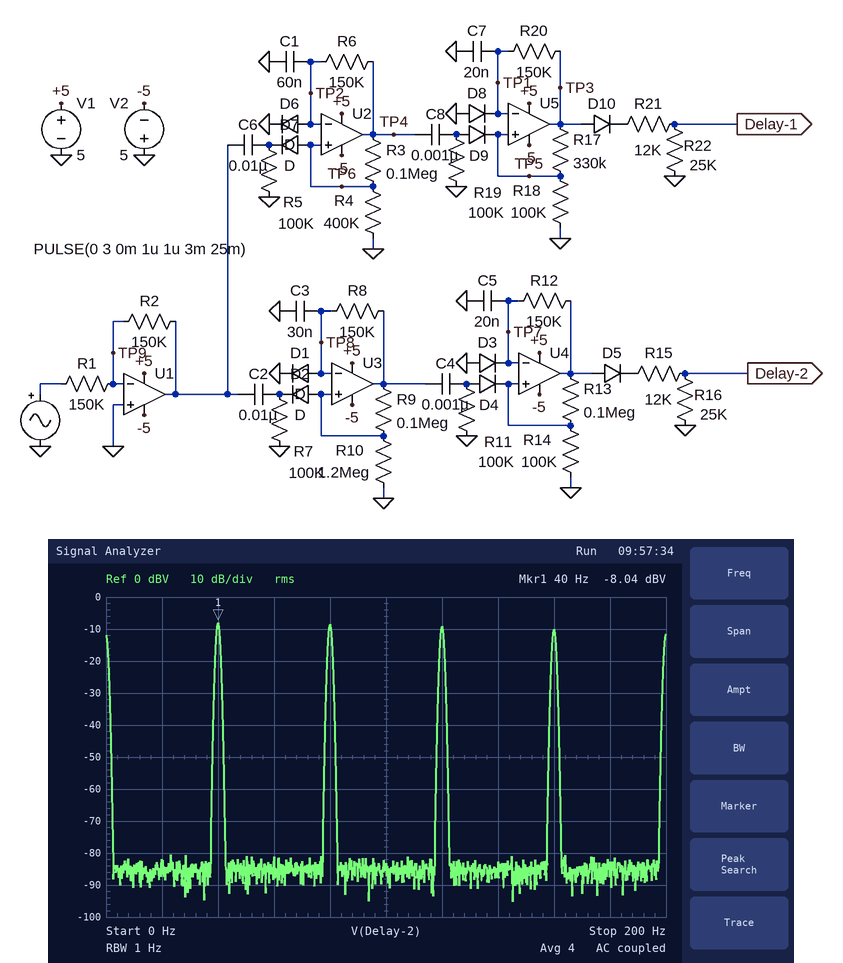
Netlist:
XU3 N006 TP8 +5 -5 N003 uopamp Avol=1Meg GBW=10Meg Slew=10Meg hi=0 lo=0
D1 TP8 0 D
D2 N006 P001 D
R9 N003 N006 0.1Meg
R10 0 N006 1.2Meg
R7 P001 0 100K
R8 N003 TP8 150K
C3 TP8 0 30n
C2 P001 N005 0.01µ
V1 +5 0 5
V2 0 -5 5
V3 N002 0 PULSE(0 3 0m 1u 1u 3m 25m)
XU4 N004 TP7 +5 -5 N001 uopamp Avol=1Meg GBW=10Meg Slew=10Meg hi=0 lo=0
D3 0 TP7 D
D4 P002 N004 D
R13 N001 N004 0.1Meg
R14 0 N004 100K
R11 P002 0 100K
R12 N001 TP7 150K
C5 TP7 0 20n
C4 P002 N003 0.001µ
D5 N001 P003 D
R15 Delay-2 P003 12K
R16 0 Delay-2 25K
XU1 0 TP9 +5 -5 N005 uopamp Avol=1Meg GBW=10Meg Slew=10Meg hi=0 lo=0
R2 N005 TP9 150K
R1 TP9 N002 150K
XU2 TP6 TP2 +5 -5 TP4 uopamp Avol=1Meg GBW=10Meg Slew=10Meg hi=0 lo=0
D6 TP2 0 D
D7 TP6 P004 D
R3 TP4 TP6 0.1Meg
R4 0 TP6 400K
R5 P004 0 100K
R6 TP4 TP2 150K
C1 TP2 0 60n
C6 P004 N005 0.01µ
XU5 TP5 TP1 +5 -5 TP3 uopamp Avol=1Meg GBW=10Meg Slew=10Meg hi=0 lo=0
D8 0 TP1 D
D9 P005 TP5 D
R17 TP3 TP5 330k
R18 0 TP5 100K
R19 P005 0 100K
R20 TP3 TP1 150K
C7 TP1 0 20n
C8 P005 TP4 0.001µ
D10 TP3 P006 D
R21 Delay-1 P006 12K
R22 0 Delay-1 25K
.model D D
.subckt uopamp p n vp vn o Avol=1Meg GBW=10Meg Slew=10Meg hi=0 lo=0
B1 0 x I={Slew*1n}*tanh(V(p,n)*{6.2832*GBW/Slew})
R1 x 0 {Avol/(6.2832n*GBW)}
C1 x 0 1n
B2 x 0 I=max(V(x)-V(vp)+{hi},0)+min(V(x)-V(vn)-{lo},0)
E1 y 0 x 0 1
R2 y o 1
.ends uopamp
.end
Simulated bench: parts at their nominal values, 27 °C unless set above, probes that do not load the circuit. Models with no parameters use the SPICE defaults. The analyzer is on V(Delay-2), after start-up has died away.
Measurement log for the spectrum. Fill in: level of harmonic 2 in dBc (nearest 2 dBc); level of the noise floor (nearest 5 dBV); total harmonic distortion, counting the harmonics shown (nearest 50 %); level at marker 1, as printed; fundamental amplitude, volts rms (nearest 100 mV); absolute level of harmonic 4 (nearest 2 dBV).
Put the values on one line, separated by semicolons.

0 dBc; -85 dBV; 150 %; -8.04 dBV; 400 mV; -10 dBV
